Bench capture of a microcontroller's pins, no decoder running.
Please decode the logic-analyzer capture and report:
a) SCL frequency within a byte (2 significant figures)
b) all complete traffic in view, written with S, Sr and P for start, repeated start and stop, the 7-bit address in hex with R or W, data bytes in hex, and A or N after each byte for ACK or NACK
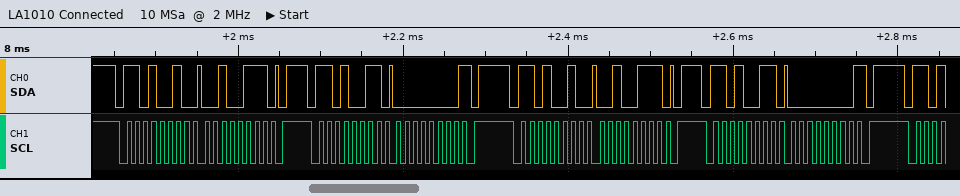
100 kHz
S 69W A 27 A P S 69R A 00 N P S 69W A 27 A P S 69R A 00 N P
